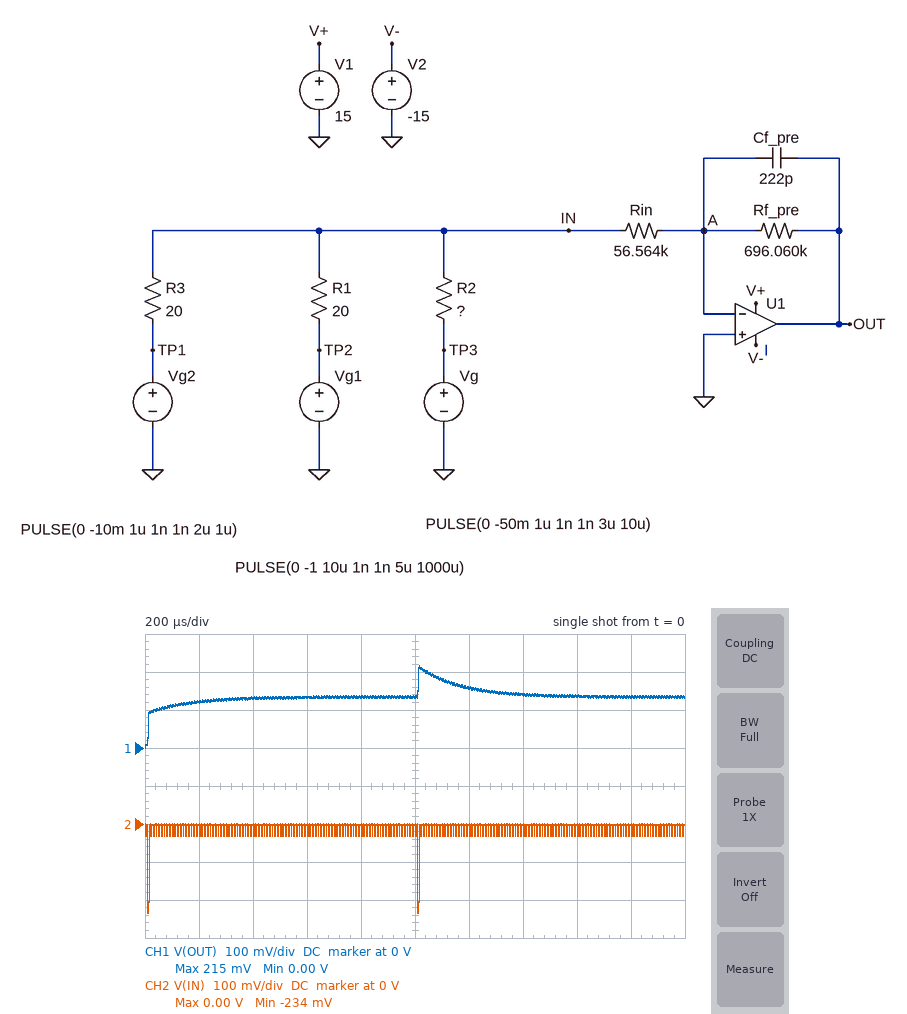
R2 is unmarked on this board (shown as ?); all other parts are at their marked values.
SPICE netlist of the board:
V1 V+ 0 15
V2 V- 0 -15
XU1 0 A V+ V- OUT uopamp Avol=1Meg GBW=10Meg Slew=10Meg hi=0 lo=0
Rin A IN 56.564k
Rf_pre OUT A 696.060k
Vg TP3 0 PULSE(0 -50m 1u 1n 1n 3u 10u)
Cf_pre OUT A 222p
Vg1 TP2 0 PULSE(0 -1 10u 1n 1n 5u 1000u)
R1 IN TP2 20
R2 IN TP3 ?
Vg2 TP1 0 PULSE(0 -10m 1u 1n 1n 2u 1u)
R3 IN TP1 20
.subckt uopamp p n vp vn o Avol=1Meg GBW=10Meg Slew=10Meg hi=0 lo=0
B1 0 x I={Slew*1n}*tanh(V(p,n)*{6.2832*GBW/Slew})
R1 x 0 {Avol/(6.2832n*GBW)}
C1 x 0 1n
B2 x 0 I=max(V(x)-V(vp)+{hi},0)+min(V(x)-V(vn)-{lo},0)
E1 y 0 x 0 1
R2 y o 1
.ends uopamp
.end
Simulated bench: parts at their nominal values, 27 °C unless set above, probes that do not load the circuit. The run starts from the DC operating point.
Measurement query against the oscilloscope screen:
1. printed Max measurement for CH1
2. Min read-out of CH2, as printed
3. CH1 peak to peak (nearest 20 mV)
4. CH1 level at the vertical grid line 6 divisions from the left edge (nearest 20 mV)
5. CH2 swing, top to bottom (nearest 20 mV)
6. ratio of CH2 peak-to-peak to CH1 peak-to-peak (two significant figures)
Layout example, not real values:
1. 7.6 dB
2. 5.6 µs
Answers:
1. 215 mV
2. -234 mV
3. 220 mV
4. 160 mV
5. 240 mV
6. 1.1
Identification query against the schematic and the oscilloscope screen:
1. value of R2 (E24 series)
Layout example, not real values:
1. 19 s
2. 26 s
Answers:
1. 6.8 Ω
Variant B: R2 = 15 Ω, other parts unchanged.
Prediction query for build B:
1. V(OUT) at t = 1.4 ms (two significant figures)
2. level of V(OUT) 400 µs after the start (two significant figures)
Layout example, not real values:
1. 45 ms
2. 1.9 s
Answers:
1. 120 mV
2. 110 mV
